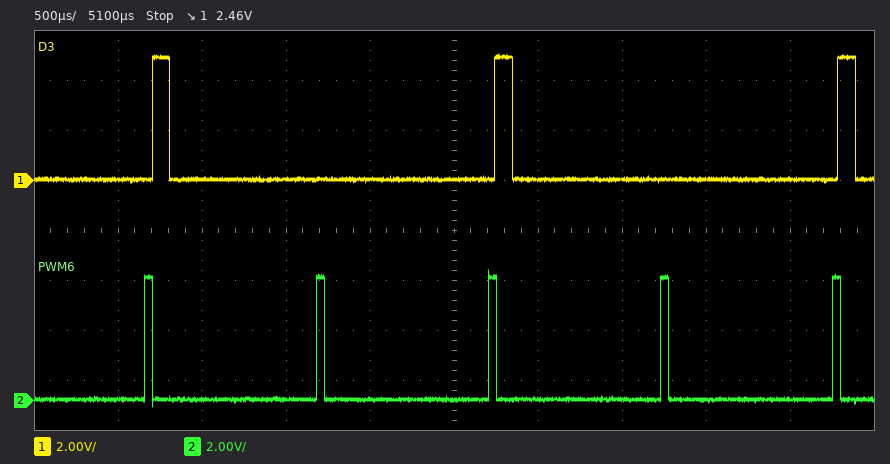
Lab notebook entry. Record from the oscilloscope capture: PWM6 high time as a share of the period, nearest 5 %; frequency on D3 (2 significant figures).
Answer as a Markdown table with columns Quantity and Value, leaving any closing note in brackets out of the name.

| Quantity | Value |
|---|---|
| PWM6 high time as a share of the period, nearest 5 % | 5 % |
| frequency on D3 | 490 Hz |
